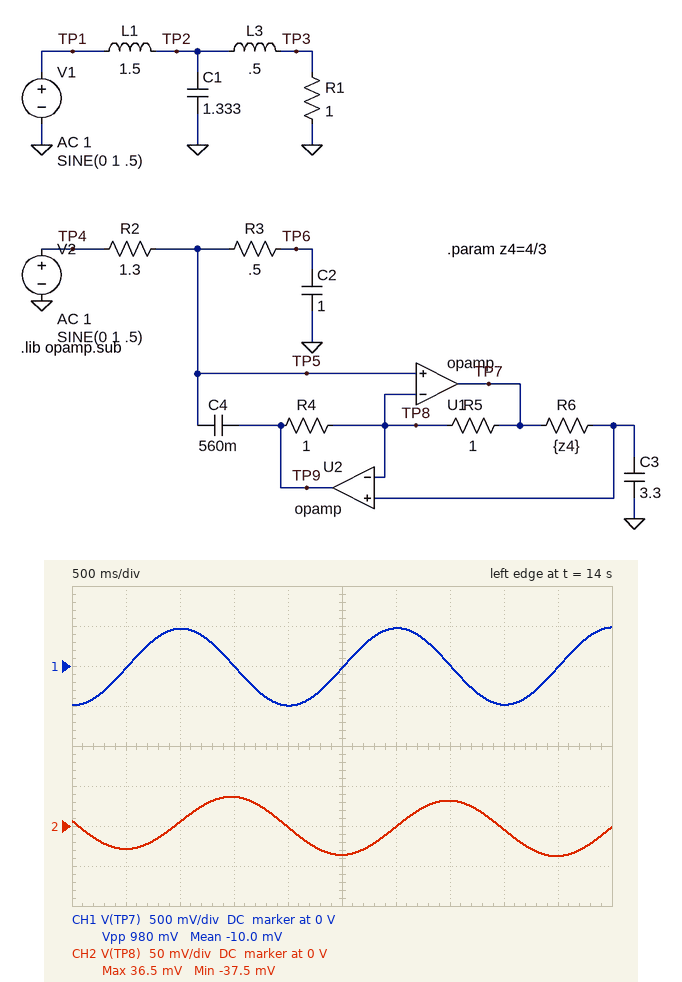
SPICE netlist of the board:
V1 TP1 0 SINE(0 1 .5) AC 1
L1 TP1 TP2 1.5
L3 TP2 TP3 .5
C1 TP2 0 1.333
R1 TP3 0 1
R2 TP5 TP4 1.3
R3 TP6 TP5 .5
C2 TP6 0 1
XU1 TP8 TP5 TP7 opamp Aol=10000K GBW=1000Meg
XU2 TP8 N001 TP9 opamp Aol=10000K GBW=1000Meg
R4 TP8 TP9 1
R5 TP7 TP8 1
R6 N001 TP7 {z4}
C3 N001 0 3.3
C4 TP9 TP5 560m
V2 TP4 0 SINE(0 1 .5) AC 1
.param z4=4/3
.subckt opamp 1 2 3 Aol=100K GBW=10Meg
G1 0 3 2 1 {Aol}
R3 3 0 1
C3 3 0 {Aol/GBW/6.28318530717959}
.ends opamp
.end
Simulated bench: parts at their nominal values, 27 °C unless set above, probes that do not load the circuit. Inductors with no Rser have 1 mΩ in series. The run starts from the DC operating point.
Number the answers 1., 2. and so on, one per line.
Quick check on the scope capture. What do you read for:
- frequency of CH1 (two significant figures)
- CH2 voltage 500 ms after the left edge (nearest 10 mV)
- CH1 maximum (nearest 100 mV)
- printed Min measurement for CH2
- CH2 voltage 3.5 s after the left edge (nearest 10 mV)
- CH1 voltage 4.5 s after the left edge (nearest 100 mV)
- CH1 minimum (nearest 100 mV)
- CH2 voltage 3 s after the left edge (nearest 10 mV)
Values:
1. 500 mHz
2. -30 mV
3. 500 mV
4. -37.5 mV
5. 30 mV
6. 0 V
7. -500 mV
8. 0 V
